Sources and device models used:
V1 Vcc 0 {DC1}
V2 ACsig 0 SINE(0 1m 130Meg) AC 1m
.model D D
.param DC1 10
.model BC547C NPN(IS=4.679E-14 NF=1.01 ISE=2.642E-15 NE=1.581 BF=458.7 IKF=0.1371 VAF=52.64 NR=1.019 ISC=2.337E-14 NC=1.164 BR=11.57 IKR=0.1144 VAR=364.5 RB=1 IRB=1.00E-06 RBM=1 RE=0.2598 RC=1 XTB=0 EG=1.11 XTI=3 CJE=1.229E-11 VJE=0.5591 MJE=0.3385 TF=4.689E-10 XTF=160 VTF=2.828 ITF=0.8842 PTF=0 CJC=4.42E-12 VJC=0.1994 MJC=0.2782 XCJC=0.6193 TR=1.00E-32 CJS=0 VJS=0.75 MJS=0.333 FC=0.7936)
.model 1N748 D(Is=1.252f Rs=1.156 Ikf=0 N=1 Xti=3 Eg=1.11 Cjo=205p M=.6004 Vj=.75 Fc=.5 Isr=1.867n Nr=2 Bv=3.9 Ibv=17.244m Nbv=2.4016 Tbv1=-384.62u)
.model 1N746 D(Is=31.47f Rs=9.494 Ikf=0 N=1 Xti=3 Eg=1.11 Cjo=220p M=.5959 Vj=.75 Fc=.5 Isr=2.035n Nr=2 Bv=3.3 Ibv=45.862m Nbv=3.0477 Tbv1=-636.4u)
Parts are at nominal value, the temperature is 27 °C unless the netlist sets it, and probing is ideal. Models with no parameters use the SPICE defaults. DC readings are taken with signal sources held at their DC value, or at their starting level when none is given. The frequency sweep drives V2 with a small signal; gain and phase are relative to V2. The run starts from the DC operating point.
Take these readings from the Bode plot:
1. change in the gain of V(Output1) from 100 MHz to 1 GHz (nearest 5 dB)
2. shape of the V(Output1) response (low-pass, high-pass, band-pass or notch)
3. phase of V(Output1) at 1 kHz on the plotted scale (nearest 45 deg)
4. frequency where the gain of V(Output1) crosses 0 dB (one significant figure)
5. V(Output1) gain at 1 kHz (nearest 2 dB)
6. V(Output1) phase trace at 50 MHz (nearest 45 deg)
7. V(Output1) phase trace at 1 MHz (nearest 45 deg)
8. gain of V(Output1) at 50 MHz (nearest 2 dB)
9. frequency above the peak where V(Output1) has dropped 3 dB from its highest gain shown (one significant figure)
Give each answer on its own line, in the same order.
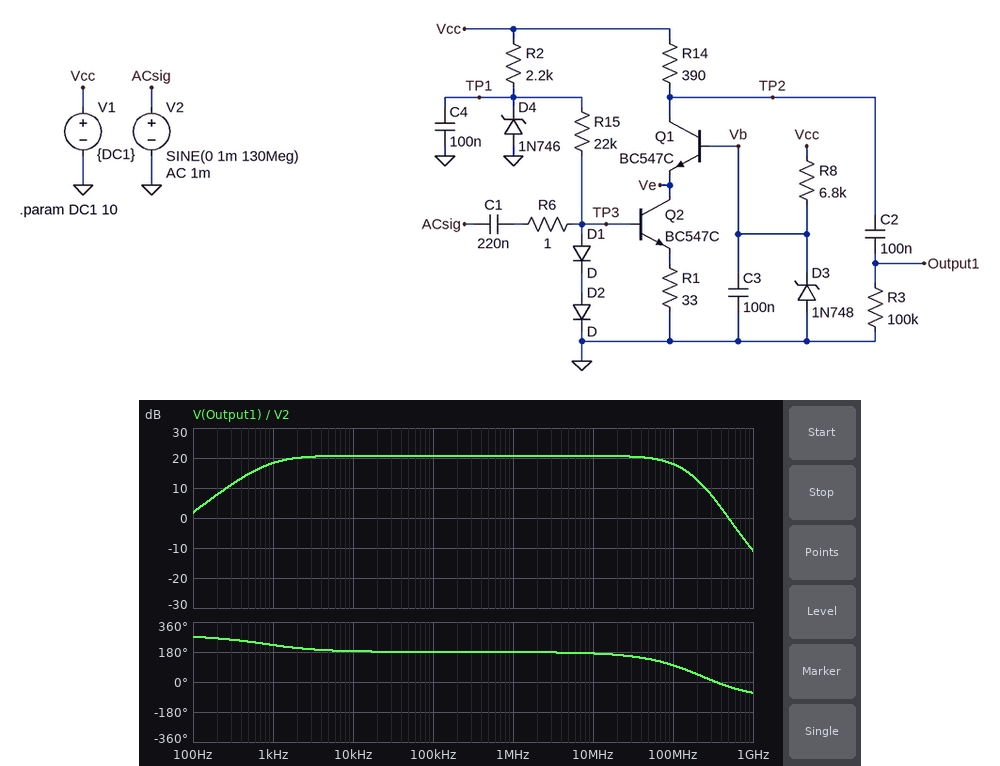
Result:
-30 dB
band-pass
225 deg
500 MHz
18 dB
135 deg
180 deg
20 dB
100 MHz
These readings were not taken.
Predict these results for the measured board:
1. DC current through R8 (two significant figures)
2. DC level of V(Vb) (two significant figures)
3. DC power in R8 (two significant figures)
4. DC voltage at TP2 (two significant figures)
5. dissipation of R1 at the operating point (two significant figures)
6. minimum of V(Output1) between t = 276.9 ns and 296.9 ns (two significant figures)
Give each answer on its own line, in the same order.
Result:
920 µA
3.7 V
5.8 mW
4.5 V
6.6 mW
-6.7 mV
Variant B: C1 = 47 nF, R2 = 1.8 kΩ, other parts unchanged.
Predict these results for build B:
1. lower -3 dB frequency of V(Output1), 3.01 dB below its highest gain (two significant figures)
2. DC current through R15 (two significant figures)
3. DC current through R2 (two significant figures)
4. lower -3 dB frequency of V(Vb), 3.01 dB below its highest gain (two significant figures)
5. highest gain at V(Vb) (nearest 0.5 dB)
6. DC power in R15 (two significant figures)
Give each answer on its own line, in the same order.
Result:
4.1 kHz
90 µA
3.8 mA
3.1 kHz
-46.5 dB
180 µW
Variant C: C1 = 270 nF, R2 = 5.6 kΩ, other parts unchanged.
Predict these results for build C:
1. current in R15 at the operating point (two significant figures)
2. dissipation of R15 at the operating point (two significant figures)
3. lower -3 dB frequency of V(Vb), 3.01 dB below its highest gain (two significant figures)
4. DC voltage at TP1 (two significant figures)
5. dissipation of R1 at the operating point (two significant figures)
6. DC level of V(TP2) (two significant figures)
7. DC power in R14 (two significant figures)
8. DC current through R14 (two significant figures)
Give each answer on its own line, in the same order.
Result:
85 µA
160 µW
630 Hz
3.0 V
6.5 mW
4.6 V
76 mW
14 mA
